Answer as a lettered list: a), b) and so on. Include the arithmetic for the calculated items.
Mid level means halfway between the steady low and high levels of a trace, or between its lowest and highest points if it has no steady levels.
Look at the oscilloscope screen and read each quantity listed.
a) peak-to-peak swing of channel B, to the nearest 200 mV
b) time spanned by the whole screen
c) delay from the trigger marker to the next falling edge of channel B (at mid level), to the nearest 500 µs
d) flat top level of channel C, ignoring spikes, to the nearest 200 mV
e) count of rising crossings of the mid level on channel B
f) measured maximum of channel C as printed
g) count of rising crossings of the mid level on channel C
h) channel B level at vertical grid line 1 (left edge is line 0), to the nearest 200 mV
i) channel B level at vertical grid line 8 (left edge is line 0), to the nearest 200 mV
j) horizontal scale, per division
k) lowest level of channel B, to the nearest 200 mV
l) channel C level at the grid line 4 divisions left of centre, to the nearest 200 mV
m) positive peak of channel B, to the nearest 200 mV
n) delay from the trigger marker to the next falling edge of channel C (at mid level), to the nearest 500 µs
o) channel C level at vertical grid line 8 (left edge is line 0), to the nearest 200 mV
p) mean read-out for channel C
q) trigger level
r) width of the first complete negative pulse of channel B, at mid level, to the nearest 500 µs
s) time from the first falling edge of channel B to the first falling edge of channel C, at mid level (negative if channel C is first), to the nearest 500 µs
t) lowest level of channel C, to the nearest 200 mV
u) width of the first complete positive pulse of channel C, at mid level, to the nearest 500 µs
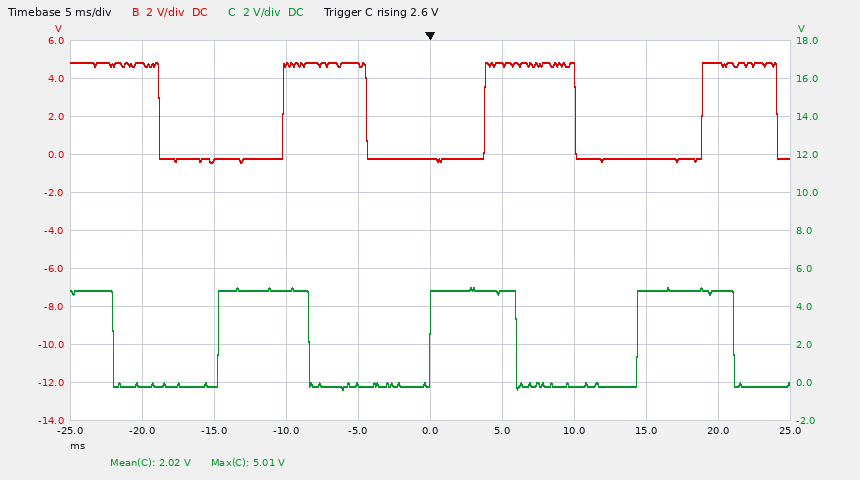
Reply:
a) 4.8 V − (-400 mV) = 5.2 V
b) 50 ms
c) 10.0 ms
d) 4.8 V
e) 3
f) 5.01 V
g) 3
h) 4.8 V
i) -200 mV
j) 5 ms
k) -400 mV
l) -200 mV
m) 4.8 V
n) 6.0 ms
o) 4.8 V
p) 2.02 V
q) 2.6 V
r) 8.5 ms
s) -3.0 ms
t) -400 mV
u) 6.5 ms
